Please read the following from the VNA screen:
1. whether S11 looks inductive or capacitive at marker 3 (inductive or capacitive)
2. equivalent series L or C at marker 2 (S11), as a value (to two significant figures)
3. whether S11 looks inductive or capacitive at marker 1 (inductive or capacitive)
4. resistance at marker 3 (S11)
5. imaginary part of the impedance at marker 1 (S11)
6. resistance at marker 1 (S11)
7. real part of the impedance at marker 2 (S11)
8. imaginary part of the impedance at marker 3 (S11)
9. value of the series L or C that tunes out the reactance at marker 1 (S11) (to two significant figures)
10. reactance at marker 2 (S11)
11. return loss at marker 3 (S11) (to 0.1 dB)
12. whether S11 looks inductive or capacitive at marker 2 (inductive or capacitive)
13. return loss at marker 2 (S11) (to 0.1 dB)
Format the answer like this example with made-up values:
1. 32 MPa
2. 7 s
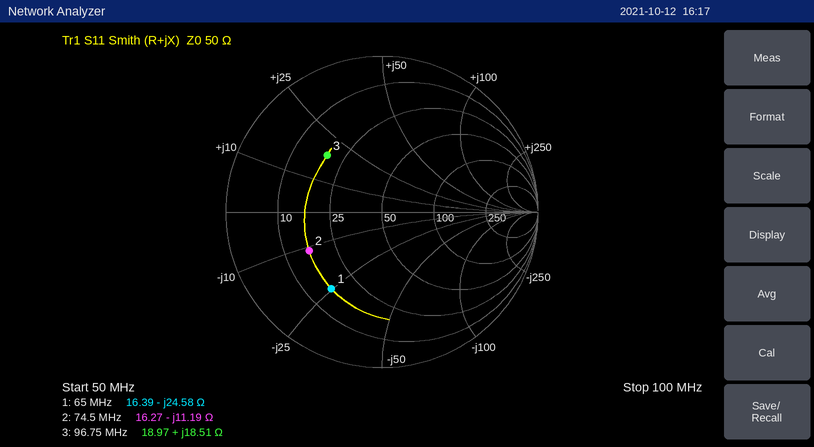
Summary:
1. inductive
2. 190 pF
3. capacitive
4. 18.97 Ω
5. -24.58 Ω
6. 16.39 Ω
7. 16.27 Ω
8. +18.51 Ω
9. 60 nH
10. -11.19 Ω
11. 5.9 dB
12. capacitive
13. 5.5 dB
